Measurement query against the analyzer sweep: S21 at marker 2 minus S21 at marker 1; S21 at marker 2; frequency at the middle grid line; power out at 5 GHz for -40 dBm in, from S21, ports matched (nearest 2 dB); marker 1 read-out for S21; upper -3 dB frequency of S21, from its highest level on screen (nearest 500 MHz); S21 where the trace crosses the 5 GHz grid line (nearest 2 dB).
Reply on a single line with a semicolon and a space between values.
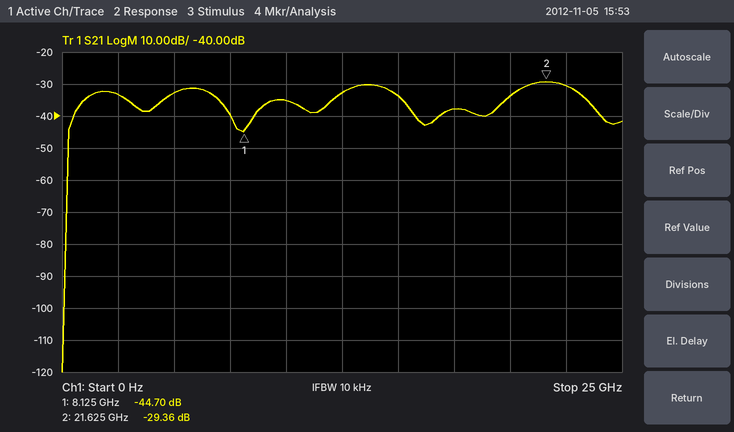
15.34 dB; -29.36 dB; 12.5 GHz; -72 dBm; -44.70 dB; 23.0 GHz; -32 dB
